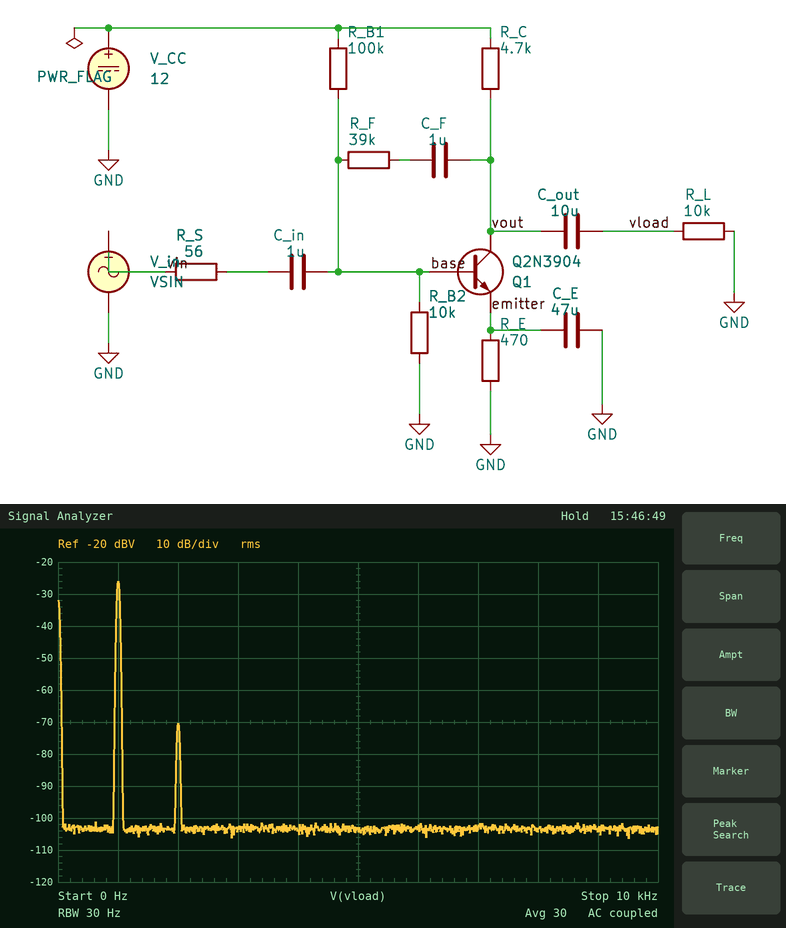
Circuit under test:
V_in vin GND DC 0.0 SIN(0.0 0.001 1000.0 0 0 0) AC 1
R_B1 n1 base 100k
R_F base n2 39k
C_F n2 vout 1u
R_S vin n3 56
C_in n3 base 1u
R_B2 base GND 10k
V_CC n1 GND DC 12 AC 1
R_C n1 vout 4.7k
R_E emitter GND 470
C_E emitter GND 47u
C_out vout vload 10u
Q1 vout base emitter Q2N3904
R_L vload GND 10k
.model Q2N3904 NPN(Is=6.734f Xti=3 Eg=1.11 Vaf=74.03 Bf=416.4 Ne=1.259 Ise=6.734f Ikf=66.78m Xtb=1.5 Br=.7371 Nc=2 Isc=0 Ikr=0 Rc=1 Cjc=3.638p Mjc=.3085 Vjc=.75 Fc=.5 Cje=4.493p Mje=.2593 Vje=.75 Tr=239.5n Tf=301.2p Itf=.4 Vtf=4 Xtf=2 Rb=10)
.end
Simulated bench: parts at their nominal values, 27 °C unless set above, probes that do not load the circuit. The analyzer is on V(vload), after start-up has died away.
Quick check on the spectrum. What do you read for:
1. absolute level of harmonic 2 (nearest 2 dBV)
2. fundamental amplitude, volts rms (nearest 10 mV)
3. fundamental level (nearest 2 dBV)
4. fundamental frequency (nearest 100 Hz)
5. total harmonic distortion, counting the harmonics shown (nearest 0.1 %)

-70 dBV
50 mV
-26 dBV
1.0 kHz
0.6 %
